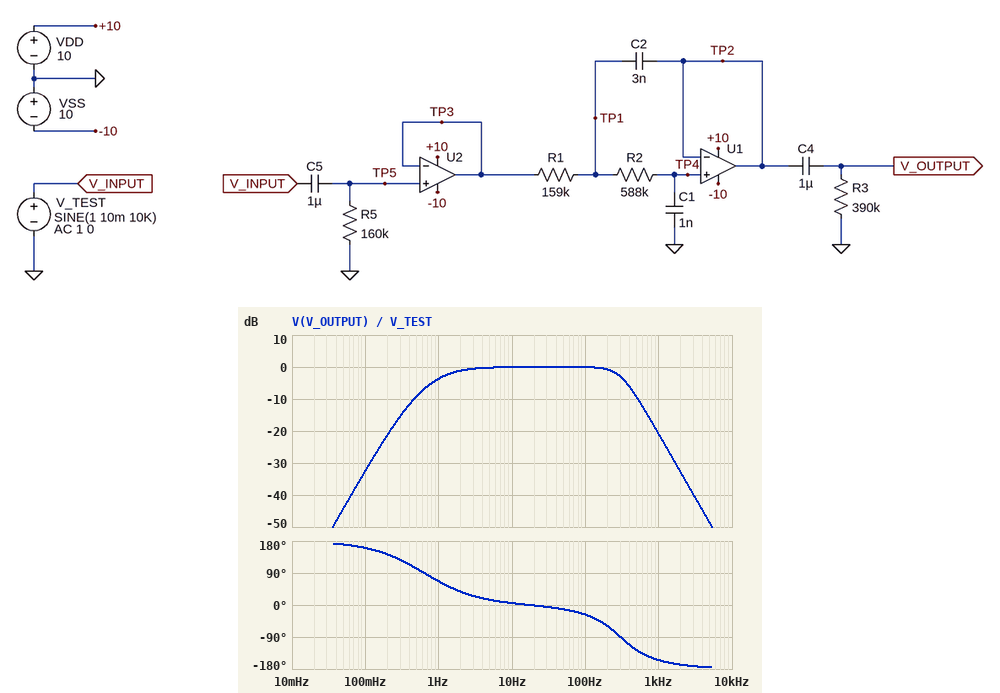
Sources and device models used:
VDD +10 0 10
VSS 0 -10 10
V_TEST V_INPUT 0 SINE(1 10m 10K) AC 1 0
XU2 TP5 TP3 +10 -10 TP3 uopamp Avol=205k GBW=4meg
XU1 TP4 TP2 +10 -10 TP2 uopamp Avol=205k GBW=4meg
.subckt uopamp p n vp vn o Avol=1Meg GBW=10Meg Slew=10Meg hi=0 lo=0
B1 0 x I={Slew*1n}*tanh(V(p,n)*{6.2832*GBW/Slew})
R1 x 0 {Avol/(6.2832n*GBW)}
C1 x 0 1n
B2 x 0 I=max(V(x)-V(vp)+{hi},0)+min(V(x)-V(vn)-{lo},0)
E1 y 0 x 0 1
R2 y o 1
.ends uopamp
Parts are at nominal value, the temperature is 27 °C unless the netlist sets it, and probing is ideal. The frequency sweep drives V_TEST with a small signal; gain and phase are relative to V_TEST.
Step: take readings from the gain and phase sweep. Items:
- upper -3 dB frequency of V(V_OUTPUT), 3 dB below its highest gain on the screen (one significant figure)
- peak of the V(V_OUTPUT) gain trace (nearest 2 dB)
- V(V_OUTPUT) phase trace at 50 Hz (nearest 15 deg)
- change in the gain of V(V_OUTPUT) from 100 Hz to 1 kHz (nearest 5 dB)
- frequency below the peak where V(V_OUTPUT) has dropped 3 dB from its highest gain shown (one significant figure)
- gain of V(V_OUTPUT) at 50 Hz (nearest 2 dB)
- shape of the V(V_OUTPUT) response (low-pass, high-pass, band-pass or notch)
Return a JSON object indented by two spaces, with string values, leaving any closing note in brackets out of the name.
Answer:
{
  "upper -3 dB frequency of V(V_OUTPUT), 3 dB below its highest gain on the screen": "300 Hz",
  "peak of the V(V_OUTPUT) gain trace": "0 dB",
  "V(V_OUTPUT) phase trace at 50 Hz": "-15 deg",
  "change in the gain of V(V_OUTPUT) from 100 Hz to 1 kHz": "-20 dB",
  "frequency below the peak where V(V_OUTPUT) has dropped 3 dB from its highest gain shown": "1 Hz",
  "gain of V(V_OUTPUT) at 50 Hz": "0 dB",
  "shape of the V(V_OUTPUT) response": "band-pass"
}
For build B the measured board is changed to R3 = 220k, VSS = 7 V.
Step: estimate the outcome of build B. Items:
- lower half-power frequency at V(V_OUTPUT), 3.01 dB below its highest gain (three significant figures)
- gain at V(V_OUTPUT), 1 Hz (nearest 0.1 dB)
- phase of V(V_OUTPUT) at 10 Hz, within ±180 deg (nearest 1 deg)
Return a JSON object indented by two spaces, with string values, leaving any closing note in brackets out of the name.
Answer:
{
  "lower half-power frequency at V(V_OUTPUT), 3.01 dB below its highest gain": "1.34 Hz",
  "gain at V(V_OUTPUT), 1 Hz": "-4.8 dB",
  "phase of V(V_OUTPUT) at 10 Hz, within ±180 deg": "7 deg"
}
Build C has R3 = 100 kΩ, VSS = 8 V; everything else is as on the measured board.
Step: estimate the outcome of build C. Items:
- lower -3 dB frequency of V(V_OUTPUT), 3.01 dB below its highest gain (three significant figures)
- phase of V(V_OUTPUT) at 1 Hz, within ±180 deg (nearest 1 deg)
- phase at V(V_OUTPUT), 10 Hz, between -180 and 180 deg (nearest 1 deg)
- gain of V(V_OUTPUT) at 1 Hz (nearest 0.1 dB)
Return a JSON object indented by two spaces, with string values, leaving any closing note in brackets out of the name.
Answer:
{
  "lower -3 dB frequency of V(V_OUTPUT), 3.01 dB below its highest gain": "2.03 Hz",
  "phase of V(V_OUTPUT) at 1 Hz, within ±180 deg": "102 deg",
  "phase at V(V_OUTPUT), 10 Hz, between -180 and 180 deg": "12 deg",
  "gain of V(V_OUTPUT) at 1 Hz": "-8.5 dB"
}
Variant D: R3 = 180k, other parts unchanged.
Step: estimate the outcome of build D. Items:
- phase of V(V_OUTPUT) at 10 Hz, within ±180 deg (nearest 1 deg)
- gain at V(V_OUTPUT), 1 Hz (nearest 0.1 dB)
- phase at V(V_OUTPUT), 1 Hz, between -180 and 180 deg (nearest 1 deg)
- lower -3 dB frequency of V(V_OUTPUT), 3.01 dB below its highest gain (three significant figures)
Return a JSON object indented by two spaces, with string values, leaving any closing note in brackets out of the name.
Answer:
{
  "phase of V(V_OUTPUT) at 10 Hz, within ±180 deg": "8 deg",
  "gain at V(V_OUTPUT), 1 Hz": "-5.5 dB",
  "phase at V(V_OUTPUT), 1 Hz, between -180 and 180 deg": "86 deg",
  "lower -3 dB frequency of V(V_OUTPUT), 3.01 dB below its highest gain": "1.46 Hz"
}
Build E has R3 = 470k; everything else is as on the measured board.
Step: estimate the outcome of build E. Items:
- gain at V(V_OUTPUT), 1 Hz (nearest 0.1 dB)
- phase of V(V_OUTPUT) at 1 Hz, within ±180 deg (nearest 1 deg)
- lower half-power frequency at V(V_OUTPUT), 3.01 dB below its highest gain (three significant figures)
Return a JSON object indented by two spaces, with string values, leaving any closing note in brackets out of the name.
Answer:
{
  "gain at V(V_OUTPUT), 1 Hz": "-3.5 dB",
  "phase of V(V_OUTPUT) at 1 Hz, within ±180 deg": "63 deg",
  "lower half-power frequency at V(V_OUTPUT), 3.01 dB below its highest gain": "1.09 Hz"
}
